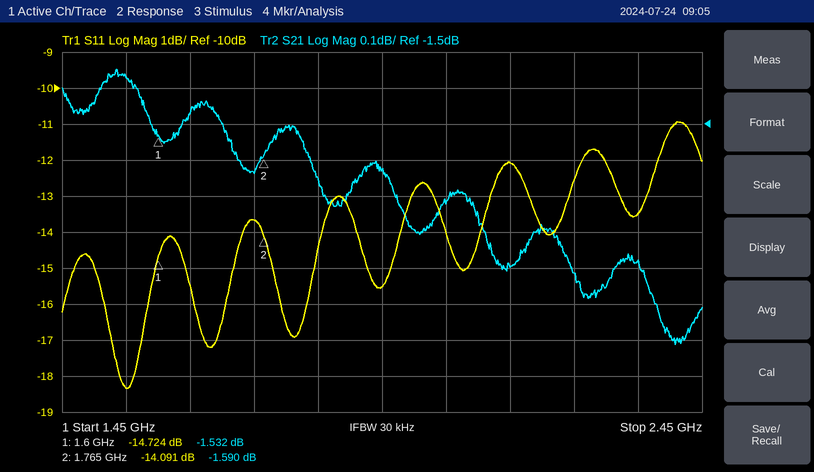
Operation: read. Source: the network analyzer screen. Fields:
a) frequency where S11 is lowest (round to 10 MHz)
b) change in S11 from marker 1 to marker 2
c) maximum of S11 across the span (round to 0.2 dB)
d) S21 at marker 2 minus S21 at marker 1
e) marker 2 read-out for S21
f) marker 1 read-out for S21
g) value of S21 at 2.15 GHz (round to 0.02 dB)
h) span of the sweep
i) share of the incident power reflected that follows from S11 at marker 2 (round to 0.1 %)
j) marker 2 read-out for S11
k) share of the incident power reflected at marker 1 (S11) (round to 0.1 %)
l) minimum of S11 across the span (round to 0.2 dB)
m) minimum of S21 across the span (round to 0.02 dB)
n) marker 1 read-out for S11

1.55 GHz
0.633 dB
-11.0 dB
-0.058 dB
-1.590 dB
-1.532 dB
-1.90 dB
1 GHz
3.9 %
-14.091 dB
3.4 %
-18.4 dB
-2.12 dB
-14.724 dB
